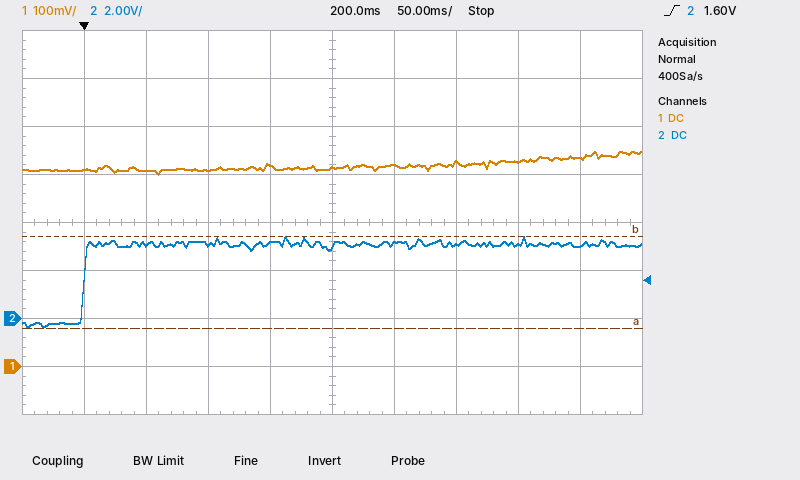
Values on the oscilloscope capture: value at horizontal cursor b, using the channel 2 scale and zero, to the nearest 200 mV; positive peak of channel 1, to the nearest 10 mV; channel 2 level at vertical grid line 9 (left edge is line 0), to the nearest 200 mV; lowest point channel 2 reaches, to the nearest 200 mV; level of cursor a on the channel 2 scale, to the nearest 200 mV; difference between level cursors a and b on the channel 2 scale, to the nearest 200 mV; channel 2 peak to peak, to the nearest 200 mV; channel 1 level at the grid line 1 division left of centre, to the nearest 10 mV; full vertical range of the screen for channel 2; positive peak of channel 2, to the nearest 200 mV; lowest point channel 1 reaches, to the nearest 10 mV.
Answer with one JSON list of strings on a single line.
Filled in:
["3.4 V", "450 mV", "3.0 V", "-400 mV", "-400 mV", "3.8 V", "3.8 V", "420 mV", "16 V", "3.4 V", "400 mV"]
